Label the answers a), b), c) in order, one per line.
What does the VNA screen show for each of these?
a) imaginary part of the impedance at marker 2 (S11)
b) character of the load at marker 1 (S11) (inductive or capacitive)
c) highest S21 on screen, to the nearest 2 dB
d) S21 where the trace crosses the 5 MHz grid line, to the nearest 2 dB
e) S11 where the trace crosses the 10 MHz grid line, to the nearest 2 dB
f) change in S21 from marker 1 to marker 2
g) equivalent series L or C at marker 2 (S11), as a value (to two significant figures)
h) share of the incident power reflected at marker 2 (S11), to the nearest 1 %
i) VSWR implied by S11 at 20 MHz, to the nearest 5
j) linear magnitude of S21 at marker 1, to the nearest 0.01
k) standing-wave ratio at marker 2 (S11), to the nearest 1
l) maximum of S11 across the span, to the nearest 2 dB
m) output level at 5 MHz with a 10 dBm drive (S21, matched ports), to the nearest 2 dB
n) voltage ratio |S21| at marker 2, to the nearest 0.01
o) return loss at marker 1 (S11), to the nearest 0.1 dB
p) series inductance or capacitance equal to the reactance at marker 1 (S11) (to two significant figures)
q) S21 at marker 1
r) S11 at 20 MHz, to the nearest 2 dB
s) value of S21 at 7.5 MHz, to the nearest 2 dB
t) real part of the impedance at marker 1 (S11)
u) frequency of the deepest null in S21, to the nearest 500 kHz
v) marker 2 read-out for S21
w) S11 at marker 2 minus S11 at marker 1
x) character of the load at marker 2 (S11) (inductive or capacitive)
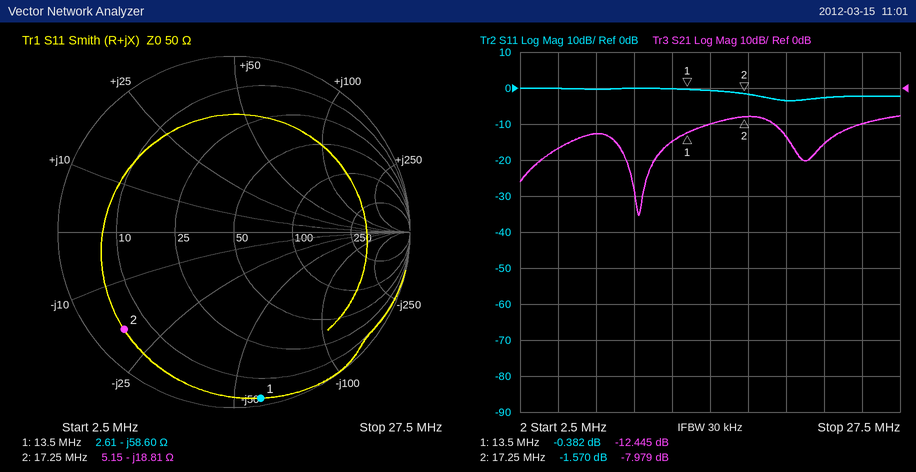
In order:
a) -18.81 Ω
b) capacitive
c) -8 dB
d) -16 dB
e) 0 dB
f) 4.466 dB
g) 490 pF
h) 70 %
i) 5
j) 0.24
k) 11
l) 0 dB
m) -6 dBm
n) 0.40
o) 0.4 dB
p) 200 pF
q) -12.445 dB
r) -4 dB
s) -12 dB
t) 2.61 Ω
u) 10.5 MHz
v) -7.979 dB
w) -1.188 dB
x) capacitive
